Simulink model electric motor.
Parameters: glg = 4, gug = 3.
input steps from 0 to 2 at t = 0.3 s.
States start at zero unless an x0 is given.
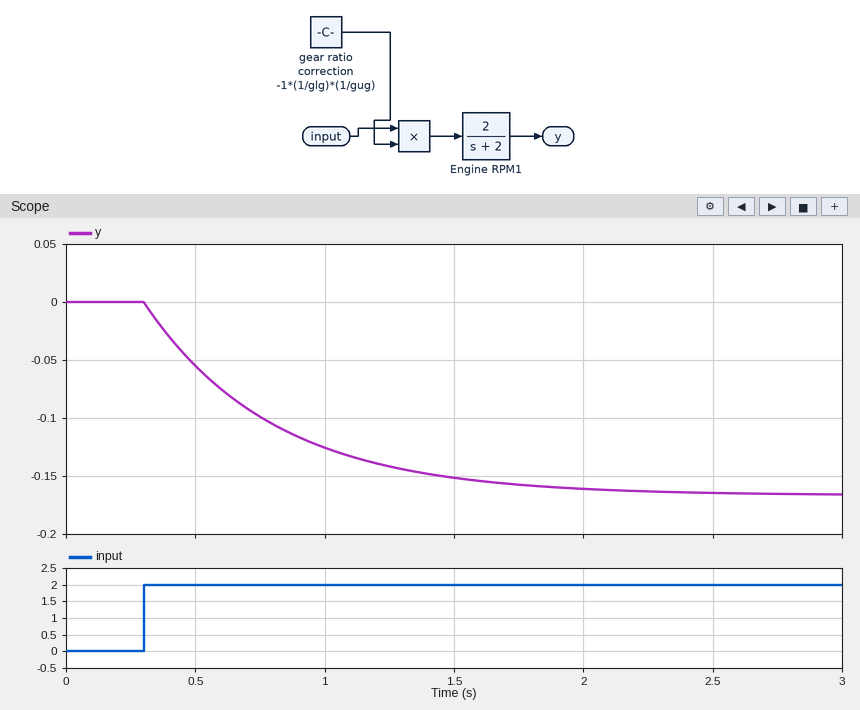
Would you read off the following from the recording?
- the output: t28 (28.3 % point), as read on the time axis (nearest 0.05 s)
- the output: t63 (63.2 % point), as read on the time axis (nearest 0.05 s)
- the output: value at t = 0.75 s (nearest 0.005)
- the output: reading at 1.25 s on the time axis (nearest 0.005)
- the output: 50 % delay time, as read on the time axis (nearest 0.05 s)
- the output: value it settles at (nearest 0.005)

0.45 s
0.80 s
-0.100
-0.140
0.65 s
-0.165
